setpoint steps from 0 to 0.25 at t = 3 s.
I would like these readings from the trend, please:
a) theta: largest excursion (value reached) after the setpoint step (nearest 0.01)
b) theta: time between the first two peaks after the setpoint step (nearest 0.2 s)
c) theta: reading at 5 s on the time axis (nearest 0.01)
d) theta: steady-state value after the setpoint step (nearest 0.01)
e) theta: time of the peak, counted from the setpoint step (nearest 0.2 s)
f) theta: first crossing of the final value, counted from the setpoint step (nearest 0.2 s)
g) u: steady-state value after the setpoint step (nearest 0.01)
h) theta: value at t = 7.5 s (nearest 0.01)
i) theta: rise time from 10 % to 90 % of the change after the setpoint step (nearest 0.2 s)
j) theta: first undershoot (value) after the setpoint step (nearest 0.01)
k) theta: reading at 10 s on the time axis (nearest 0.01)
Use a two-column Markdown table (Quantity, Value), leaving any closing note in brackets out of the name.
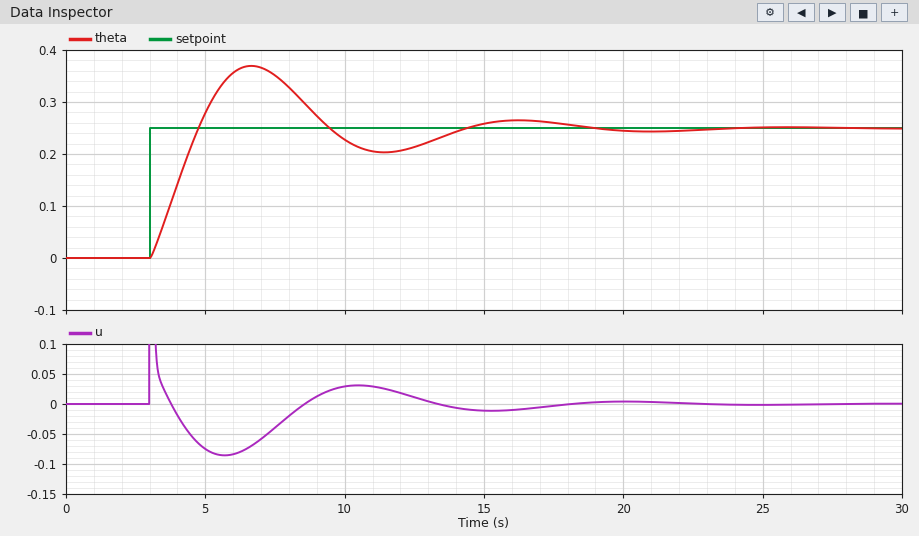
| Quantity | Value |
|---|---|
| theta: largest excursion (value reached) after the setpoint step | 0.37 |
| theta: time between the first two peaks after the setpoint step | 9.6 s |
| theta: reading at 5 s on the time axis | 0.28 |
| theta: steady-state value after the setpoint step | 0.25 |
| theta: time of the peak, counted from the setpoint step | 3.6 s |
| theta: first crossing of the final value, counted from the setpoint step | 1.8 s |
| u: steady-state value after the setpoint step | 0.00 |
| theta: value at t = 7.5 s | 0.35 |
| theta: rise time from 10 % to 90 % of the change after the setpoint step | 1.4 s |
| theta: first undershoot (value) after the setpoint step | 0.20 |
| theta: reading at 10 s on the time axis | 0.23 |
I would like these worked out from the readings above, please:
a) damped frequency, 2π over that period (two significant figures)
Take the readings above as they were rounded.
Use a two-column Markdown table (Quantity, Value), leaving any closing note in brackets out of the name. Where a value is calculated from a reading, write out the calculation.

| Quantity | Value |
|---|---|
| damped frequency, 2π over that period | 2π / 9.6 = 0.65 rad/s |
